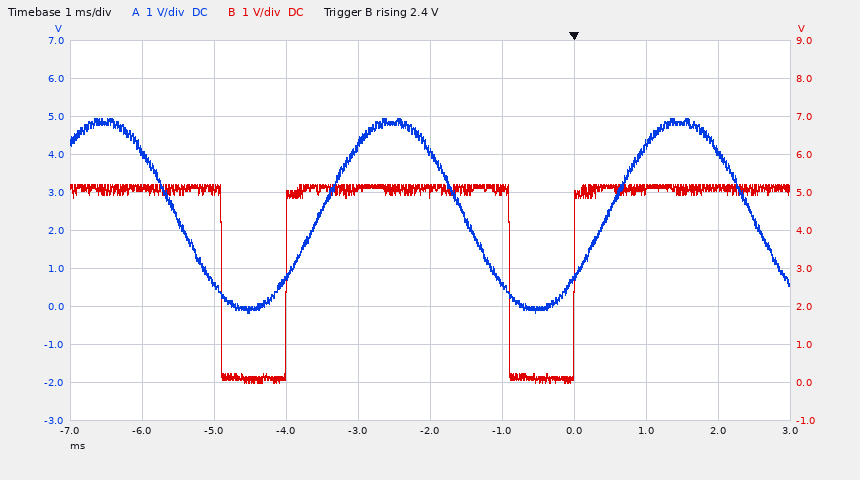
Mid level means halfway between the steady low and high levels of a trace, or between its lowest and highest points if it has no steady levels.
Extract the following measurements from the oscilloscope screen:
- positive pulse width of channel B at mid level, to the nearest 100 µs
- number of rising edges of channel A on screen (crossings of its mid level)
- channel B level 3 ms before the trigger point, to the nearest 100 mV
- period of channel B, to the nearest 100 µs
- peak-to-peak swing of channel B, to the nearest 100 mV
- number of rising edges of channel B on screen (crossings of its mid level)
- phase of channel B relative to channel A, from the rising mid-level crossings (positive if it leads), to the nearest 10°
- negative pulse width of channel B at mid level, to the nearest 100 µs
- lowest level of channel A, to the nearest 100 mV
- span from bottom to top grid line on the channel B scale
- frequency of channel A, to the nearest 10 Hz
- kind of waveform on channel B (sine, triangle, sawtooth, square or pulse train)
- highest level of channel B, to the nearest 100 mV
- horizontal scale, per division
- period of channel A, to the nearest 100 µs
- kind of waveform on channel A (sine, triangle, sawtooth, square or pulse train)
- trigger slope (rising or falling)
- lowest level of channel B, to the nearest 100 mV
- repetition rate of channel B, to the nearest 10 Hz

3.1 ms
2
5.1 V
4.0 ms
5.2 V
2
+40°
900 µs
-200 mV
10 V
250 Hz
pulse train
5.2 V
1 ms
4.0 ms
sine
rising
0.0 V
250 Hz
